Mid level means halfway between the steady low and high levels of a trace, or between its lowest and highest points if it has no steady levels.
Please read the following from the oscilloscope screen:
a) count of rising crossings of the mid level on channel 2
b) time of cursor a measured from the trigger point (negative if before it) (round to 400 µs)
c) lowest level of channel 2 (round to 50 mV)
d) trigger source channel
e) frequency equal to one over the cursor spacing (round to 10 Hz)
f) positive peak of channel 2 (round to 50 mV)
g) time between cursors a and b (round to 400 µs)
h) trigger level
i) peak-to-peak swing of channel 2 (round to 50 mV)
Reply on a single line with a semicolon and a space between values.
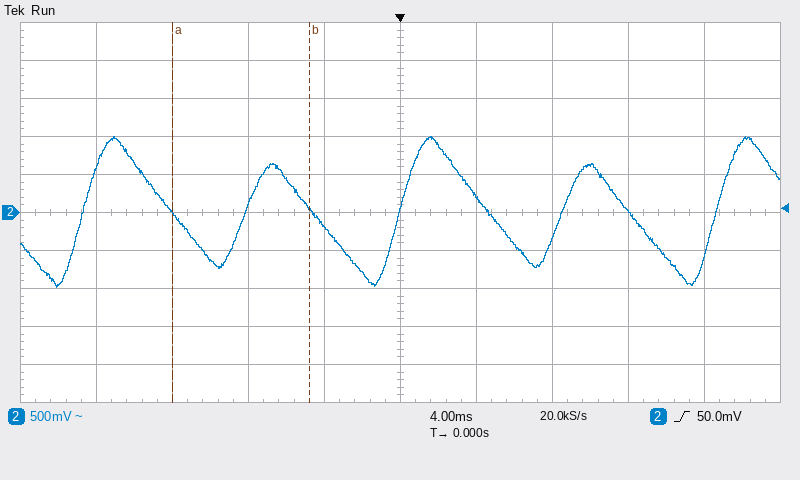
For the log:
5; -12.0 ms; -1.00 V; channel 2; 140 Hz; 1.00 V; 7.2 ms; 50.0 mV; 2.00 V
